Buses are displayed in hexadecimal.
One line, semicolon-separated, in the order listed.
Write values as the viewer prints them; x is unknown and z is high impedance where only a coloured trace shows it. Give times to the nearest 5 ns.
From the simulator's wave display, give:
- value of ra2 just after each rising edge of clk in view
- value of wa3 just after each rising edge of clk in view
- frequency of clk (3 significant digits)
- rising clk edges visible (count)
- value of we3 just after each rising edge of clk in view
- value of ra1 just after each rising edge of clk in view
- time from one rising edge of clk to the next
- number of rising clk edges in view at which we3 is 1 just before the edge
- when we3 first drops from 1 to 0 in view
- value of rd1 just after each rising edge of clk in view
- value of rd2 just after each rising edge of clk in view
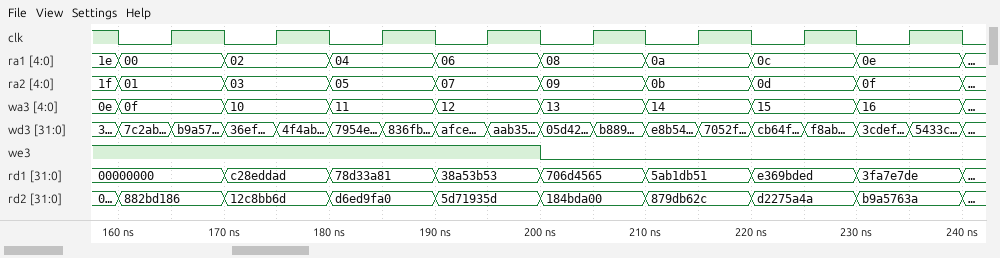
01, 03, 05, 07, 09, 0b, 0d, 0f; 0f, 10, 11, 12, 13, 14, 15, 16; 100 MHz; 8; 1 1 1 1 0 0 0 0; 00, 02, 04, 06, 08, 0a, 0c, 0e; 10 ns; 4; 200 ns; 00000000, c28eddad, 78d33a81, 38a53b53, 706d4565, 5ab1db51, e369bded, 3fa7e7de; 882bd186, 12c8bb6d, d6ed9fa0, 5d71935d, 184bda00, 879db62c, d2275a4a, b9a5763a
